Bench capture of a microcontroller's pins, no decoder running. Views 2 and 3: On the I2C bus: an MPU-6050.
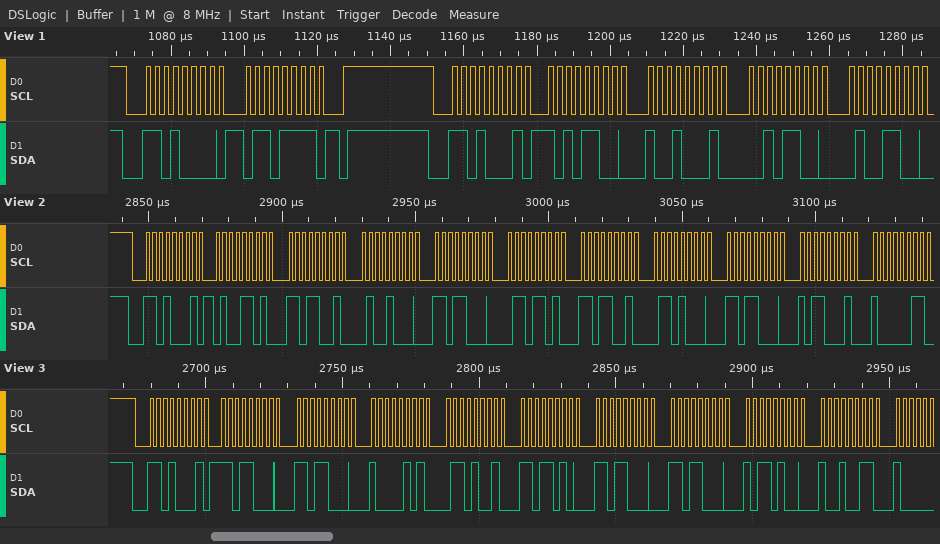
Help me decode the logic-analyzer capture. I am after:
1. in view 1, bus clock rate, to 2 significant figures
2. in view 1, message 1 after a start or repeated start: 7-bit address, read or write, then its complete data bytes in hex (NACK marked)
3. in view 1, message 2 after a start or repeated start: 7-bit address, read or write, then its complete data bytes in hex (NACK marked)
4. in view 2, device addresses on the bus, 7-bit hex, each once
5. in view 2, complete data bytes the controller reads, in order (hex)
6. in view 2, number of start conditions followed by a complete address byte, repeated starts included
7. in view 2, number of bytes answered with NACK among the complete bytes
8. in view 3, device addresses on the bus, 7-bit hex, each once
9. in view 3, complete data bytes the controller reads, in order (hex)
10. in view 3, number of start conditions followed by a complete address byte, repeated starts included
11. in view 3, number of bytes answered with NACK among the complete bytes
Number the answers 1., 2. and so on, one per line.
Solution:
1. 400 kHz
2. 0x68 write: 6F
3. 0x68 read: AC 91 2C 4C
4. 0x68
5. 4D D9 48 D8 6D D9 68 D8 B1 83
6. 1
7. 0
8. 0x68
9. D8 D8 85 69 DA D8 D8 B4 93
10. 1
11. 0
